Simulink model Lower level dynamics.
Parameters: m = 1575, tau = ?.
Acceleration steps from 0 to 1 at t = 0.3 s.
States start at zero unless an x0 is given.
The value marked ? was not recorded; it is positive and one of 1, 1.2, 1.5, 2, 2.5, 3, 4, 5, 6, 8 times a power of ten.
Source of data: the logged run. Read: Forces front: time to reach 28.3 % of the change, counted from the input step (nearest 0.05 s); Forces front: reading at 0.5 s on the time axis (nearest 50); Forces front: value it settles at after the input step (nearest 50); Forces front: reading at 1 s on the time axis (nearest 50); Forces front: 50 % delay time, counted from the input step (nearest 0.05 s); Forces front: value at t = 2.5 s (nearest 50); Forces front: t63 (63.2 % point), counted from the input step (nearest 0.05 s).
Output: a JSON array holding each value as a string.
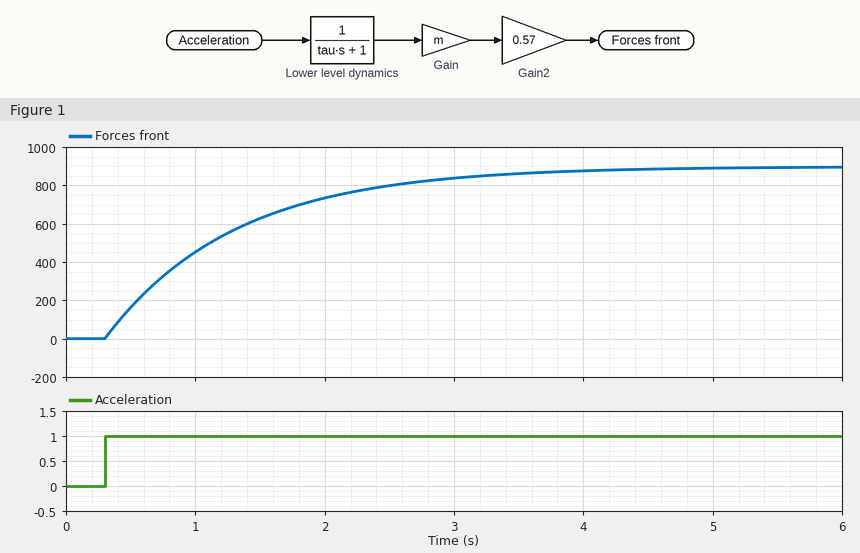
["0.35 s", "150", "900", "450", "0.70 s", "800", "1.00 s"]
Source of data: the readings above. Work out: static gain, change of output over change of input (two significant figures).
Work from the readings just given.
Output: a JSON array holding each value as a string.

["900"]
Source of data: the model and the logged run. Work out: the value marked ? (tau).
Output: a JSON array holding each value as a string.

["1"]
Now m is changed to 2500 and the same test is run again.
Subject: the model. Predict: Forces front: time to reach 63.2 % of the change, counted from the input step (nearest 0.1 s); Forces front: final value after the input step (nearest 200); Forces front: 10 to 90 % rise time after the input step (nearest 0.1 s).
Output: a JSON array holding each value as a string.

["1.0 s", "1400", "2.2 s"]
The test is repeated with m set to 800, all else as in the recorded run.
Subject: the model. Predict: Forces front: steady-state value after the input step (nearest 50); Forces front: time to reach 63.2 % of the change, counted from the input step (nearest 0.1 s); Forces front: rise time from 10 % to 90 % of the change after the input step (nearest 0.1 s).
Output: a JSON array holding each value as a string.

["450", "1.0 s", "2.2 s"]
